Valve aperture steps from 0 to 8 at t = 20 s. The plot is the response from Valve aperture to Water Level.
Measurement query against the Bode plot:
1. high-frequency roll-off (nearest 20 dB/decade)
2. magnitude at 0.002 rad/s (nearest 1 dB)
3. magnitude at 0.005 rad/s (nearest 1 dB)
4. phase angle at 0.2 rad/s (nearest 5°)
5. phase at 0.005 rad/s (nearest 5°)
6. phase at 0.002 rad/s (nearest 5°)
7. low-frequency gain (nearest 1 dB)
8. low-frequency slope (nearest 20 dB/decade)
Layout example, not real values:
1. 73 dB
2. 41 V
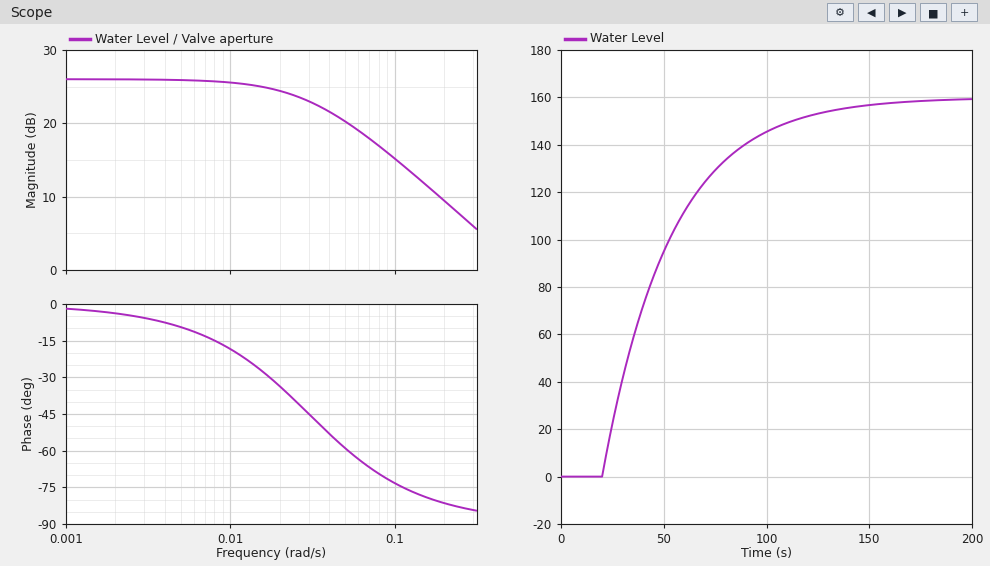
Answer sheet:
1. -20 dB/decade
2. 26 dB
3. 26 dB
4. -80°
5. -10°
6. -5°
7. 26 dB
8. 0 dB/decade
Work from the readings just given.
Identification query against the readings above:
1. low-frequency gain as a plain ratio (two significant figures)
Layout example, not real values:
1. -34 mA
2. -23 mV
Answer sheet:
1. 20
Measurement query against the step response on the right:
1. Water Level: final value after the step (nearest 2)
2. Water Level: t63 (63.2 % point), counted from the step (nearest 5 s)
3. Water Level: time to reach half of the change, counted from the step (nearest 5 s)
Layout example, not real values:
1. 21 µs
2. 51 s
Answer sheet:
1. 160
2. 35 s
3. 25 s
